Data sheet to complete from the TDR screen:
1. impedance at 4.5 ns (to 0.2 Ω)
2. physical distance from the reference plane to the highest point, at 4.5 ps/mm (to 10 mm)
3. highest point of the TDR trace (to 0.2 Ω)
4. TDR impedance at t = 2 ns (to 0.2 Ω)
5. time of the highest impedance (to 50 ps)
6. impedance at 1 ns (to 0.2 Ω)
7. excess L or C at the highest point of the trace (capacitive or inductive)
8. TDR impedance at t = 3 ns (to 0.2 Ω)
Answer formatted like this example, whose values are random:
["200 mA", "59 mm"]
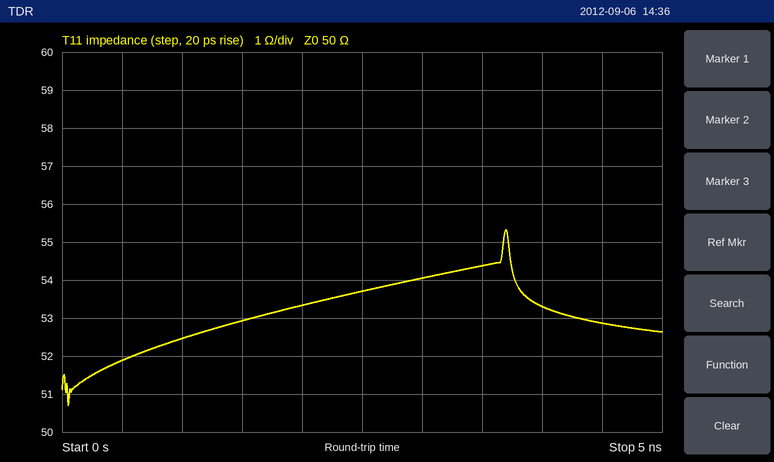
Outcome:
["52.8 Ω", "410 mm", "55.4 Ω", "53.4 Ω", "3.70 ns", "52.4 Ω", "inductive", "54.0 Ω"]
